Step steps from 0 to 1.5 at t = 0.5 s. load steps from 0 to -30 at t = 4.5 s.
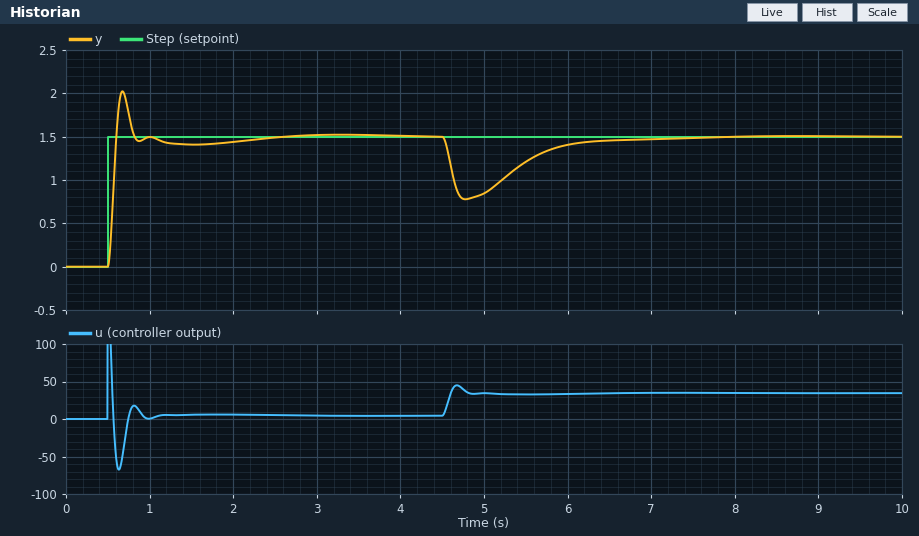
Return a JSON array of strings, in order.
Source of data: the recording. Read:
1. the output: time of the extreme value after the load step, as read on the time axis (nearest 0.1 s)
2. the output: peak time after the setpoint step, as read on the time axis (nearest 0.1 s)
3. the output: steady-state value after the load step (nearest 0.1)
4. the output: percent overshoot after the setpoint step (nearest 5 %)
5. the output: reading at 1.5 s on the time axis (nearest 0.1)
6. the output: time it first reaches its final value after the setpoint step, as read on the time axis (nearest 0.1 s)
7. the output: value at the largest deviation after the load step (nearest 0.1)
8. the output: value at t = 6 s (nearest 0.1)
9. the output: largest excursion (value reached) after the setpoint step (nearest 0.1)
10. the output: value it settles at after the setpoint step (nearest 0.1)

["4.8 s", "0.7 s", "1.5", "35 %", "1.4", "0.6 s", "0.8", "1.4", "2.0", "1.5"]
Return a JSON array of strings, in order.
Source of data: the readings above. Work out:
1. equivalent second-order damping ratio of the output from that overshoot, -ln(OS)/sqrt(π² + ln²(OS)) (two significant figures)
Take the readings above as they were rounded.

["0.32"]
